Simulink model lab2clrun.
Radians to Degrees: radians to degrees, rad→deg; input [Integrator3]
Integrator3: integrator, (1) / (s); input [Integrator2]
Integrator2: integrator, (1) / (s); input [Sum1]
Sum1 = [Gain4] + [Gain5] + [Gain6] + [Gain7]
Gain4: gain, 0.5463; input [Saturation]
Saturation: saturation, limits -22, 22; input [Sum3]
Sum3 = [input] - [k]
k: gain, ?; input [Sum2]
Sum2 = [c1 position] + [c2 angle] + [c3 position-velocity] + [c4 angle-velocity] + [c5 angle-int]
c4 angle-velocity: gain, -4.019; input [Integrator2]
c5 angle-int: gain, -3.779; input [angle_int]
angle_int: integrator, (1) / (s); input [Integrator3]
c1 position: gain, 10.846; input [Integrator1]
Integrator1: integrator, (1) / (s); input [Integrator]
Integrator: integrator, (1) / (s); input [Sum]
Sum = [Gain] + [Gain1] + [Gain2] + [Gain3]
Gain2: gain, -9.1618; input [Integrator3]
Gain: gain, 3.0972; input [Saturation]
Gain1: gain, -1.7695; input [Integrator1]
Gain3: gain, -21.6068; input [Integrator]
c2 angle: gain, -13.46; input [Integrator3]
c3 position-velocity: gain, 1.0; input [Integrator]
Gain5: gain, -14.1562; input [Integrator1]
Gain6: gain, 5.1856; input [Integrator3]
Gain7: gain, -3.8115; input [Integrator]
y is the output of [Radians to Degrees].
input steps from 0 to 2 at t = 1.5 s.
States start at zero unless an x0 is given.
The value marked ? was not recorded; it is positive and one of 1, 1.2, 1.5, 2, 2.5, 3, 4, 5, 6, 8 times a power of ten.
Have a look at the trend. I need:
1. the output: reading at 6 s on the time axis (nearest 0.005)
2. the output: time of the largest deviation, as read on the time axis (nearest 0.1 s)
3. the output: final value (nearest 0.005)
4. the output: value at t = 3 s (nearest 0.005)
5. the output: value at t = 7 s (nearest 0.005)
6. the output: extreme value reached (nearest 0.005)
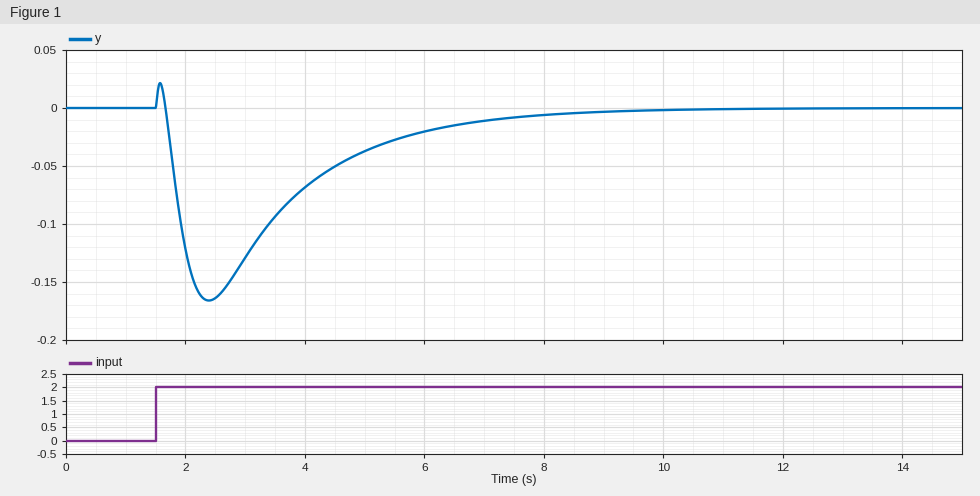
-0.020
2.4 s
0.000
-0.130
-0.010
-0.165
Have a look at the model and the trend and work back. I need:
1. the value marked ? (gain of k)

80
